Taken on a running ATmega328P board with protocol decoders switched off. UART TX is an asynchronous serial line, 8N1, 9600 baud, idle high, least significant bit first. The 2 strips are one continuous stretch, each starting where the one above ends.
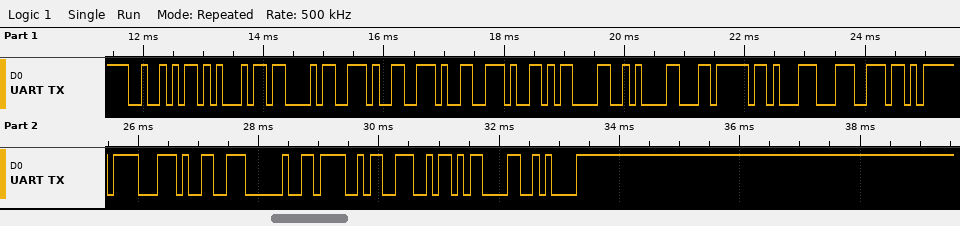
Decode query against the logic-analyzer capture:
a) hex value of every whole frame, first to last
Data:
0x52 0x45 0x43 0x2E 0x2E 0x2E 0x0D 0x0A 0xEC 0x8B 0x9C 0xEB 0x8F 0x99 0x20 0x4F 0x4E 0x0D 0x0A
